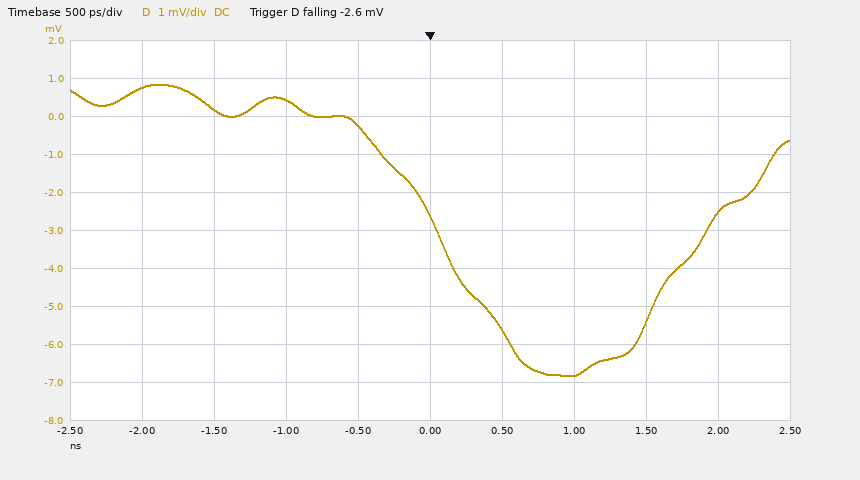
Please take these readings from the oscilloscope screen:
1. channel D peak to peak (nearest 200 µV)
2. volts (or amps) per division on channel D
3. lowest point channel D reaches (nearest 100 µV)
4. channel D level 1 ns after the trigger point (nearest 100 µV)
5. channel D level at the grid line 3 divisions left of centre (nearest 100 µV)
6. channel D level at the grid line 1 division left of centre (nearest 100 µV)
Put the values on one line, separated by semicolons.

7.6 mV; 1 mV; -6.8 mV; -6.8 mV; 200 µV; -200 µV
